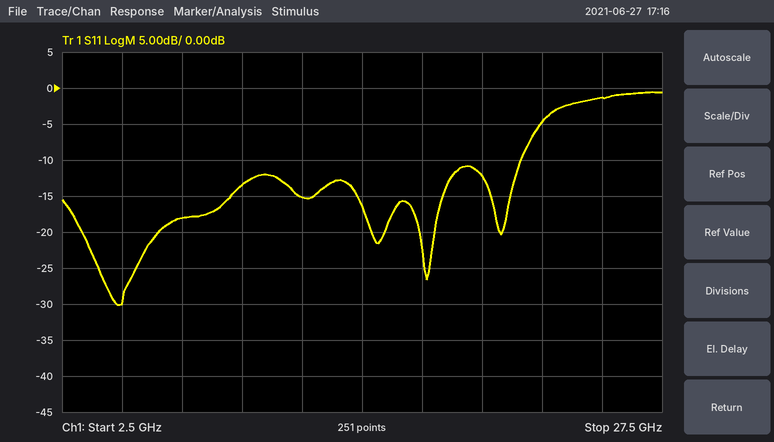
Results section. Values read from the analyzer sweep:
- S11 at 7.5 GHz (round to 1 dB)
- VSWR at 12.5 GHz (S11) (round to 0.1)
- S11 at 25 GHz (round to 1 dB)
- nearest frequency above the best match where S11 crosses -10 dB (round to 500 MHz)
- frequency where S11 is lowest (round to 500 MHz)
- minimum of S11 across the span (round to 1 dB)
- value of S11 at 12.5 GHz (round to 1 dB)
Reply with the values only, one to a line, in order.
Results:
-18 dB
1.4
-1 dB
21.5 GHz
5.0 GHz
-30 dB
-15 dB
